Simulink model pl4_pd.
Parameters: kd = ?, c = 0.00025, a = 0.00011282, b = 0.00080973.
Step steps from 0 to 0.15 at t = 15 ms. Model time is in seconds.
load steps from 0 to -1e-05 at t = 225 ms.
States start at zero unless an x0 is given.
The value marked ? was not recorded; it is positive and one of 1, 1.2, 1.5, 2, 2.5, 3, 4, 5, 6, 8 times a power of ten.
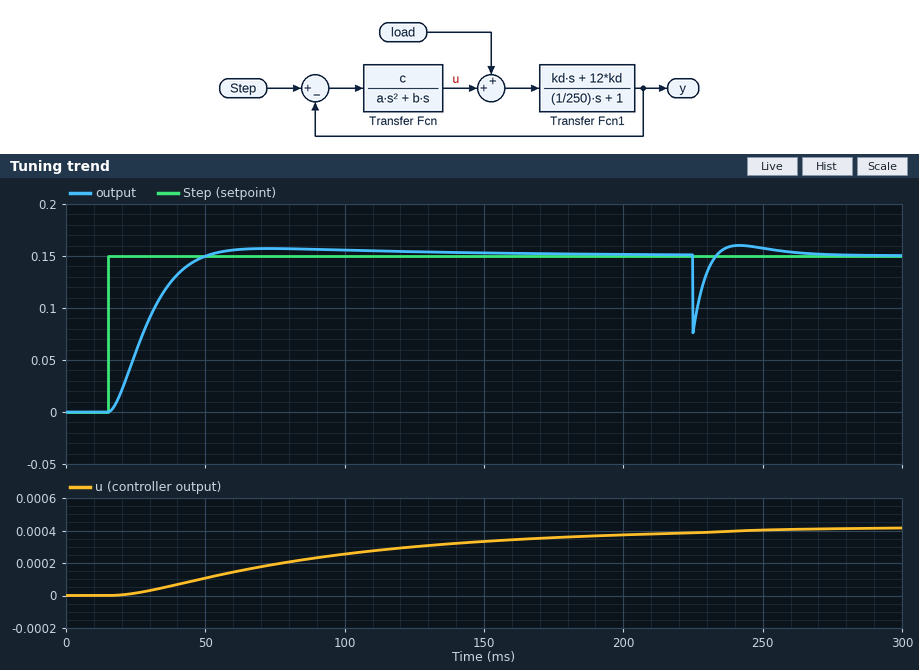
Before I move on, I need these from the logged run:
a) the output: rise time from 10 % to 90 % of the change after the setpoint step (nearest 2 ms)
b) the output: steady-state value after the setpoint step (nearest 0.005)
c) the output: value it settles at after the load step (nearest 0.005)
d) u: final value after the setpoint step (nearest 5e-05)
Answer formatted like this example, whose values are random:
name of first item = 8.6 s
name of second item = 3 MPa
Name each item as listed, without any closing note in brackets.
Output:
the output: rise time from 10 % to 90 % of the change after the setpoint step = 22 ms
the output: steady-state value after the setpoint step = 0.150
the output: value it settles at after the load step = 0.150
u: final value after the setpoint step = 0.00040
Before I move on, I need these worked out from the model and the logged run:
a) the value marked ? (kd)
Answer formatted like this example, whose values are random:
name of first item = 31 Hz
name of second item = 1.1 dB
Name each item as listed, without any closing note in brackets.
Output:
the value marked ? = 30
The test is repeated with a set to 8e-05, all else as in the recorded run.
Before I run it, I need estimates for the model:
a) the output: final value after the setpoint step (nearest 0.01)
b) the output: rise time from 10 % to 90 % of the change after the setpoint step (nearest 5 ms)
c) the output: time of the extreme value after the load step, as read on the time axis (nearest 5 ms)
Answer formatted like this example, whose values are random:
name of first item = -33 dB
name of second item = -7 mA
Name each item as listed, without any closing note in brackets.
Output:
the output: final value after the setpoint step = 0.15
the output: rise time from 10 % to 90 % of the change after the setpoint step = 15 ms
the output: time of the extreme value after the load step, as read on the time axis = 225 ms
